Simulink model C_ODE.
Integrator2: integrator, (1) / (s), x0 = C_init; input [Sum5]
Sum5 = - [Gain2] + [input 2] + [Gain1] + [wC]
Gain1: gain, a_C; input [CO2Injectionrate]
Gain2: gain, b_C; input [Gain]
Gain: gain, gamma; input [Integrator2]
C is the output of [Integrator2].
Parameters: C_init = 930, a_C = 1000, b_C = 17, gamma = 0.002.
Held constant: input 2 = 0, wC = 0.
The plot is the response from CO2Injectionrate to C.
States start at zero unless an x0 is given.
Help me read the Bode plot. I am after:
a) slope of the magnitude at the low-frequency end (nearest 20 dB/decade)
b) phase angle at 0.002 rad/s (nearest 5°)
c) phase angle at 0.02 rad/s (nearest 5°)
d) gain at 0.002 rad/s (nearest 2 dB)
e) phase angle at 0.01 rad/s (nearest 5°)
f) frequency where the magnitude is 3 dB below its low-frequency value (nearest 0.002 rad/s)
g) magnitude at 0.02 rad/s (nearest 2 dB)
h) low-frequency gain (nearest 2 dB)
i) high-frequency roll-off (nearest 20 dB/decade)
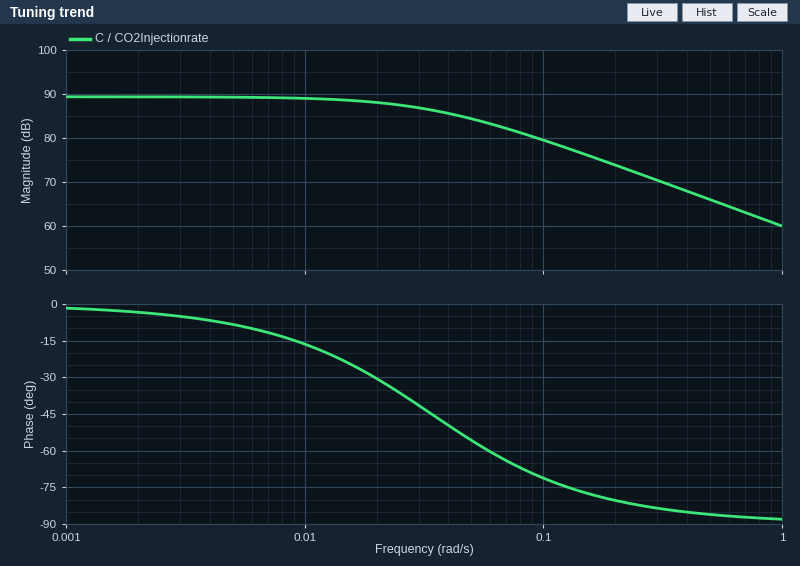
0 dB/decade
-5°
-30°
90 dB
-15°
0.034 rad/s
88 dB
90 dB
-20 dB/decade
